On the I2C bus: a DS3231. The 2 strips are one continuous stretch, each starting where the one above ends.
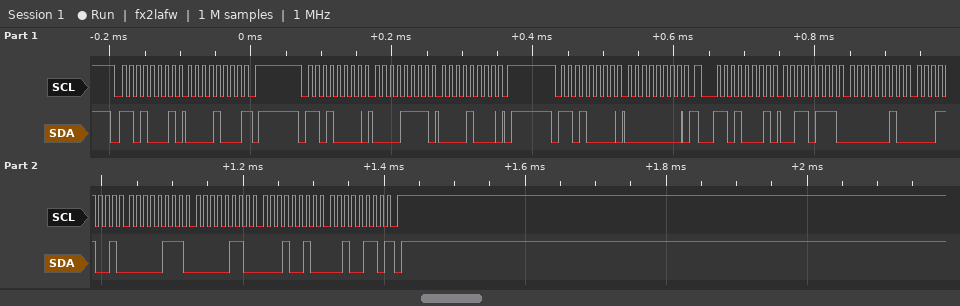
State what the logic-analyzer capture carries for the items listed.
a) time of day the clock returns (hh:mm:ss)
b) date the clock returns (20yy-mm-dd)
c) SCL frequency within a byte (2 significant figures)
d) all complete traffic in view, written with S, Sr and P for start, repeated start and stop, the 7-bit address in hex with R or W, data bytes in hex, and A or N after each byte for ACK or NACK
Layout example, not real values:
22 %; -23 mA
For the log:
19:02:37; 2026-12-06; 100 kHz; S 68R A 08 N P S 68W A 0F A 08 A P S 68W A 00 A Sr 68R A 37 A 02 A 19 A 07 A 06 A 12 A 26 N P
